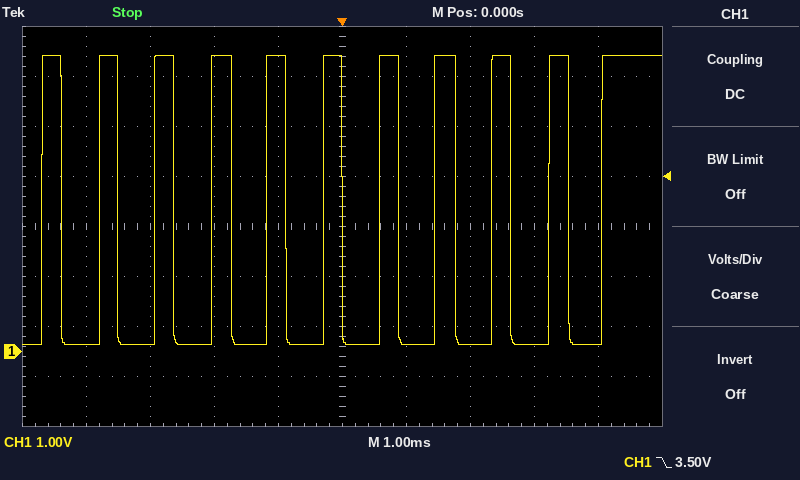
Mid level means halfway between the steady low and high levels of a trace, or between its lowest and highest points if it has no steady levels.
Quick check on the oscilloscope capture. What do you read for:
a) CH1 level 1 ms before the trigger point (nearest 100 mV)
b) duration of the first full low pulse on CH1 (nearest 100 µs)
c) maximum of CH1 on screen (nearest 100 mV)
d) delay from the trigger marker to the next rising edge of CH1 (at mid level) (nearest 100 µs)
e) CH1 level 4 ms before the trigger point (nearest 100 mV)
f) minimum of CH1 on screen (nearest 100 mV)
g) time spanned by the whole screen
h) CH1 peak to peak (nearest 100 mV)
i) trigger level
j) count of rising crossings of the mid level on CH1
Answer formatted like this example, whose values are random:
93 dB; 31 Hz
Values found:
5.9 V; 600 µs; 5.9 V; 600 µs; 100 mV; 100 mV; 10 ms; 5.8 V; 3.50 V; 11
